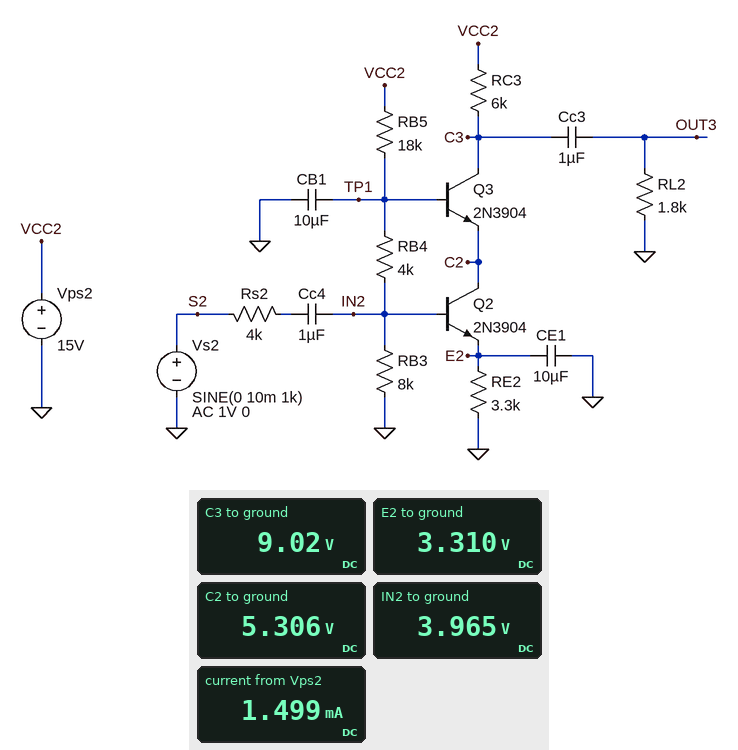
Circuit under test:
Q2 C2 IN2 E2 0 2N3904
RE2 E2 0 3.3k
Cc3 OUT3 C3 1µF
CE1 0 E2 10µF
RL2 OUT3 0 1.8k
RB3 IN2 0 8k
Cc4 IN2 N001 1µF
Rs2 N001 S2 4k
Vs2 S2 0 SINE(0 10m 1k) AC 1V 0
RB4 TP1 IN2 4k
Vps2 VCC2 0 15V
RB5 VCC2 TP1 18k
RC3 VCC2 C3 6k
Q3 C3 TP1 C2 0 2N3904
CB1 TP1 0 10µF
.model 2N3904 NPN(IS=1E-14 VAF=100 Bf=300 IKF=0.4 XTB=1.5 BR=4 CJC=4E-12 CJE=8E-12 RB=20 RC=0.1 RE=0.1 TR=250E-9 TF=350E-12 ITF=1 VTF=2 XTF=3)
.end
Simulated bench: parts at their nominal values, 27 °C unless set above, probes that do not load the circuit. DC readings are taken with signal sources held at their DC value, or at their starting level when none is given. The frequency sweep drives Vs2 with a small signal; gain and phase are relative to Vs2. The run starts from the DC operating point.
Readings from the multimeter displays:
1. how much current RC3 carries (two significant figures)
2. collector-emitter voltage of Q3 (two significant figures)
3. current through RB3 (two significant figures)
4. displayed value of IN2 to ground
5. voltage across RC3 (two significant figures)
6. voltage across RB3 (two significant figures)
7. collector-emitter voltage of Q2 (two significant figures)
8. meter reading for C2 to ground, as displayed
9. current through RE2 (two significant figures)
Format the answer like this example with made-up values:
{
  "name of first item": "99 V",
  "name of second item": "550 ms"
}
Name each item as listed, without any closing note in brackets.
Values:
{
  "how much current RC3 carries": "1.0 mA",
  "collector-emitter voltage of Q3": "3.7 V",
  "current through RB3": "500 µA",
  "displayed value of IN2 to ground": "3.965 V",
  "voltage across RC3": "6.0 V",
  "voltage across RB3": "4.0 V",
  "collector-emitter voltage of Q2": "2.0 V",
  "meter reading for C2 to ground, as displayed": "5.306 V",
  "current through RE2": "1.0 mA"
}
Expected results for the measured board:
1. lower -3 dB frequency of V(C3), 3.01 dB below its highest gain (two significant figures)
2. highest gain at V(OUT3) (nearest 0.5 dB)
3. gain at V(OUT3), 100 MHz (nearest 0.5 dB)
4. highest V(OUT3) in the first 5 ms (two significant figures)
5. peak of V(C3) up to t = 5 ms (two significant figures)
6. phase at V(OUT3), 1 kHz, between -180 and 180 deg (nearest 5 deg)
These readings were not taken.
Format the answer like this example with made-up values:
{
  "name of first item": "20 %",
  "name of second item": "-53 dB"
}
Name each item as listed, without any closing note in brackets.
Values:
{
  "lower -3 dB frequency of V(C3), 3.01 dB below its highest gain": "500 Hz",
  "highest gain at V(OUT3)": "25.0 dB",
  "gain at V(OUT3), 100 MHz": "-12.0 dB",
  "highest V(OUT3) in the first 5 ms": "160 mV",
  "peak of V(C3) up to t = 5 ms": "9.2 V",
  "phase at V(OUT3), 1 kHz, between -180 and 180 deg": "-150 deg"
}
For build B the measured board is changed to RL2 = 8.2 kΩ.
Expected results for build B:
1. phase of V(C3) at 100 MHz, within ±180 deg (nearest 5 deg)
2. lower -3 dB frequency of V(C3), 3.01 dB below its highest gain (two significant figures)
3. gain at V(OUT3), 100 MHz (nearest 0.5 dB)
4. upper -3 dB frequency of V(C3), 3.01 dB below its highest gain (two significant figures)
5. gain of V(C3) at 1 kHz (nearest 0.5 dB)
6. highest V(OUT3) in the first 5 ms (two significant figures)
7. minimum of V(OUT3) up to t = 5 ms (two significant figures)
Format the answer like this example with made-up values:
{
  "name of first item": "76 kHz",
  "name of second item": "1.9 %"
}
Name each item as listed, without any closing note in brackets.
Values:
{
  "phase of V(C3) at 100 MHz, within ±180 deg": "-15 deg",
  "lower -3 dB frequency of V(C3), 3.01 dB below its highest gain": "520 Hz",
  "gain at V(OUT3), 100 MHz": "-11.5 dB",
  "upper -3 dB frequency of V(C3), 3.01 dB below its highest gain": "3.6 MHz",
  "gain of V(C3) at 1 kHz": "32.0 dB",
  "highest V(OUT3) in the first 5 ms": "400 mV",
  "minimum of V(OUT3) up to t = 5 ms": "-400 mV"
}
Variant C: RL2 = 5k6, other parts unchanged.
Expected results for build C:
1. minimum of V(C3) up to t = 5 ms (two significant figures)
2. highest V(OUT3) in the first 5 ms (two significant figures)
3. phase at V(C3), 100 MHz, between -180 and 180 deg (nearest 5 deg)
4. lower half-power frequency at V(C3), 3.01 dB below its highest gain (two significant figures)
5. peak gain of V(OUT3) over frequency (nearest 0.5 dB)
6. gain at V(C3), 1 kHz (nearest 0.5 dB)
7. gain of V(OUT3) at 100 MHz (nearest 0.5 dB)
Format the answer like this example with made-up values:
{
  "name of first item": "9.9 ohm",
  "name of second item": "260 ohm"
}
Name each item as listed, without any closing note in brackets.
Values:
{
  "minimum of V(C3) up to t = 5 ms": "8.7 V",
  "highest V(OUT3) in the first 5 ms": "330 mV",
  "phase at V(C3), 100 MHz, between -180 and 180 deg": "-10 deg",
  "lower half-power frequency at V(C3), 3.01 dB below its highest gain": "520 Hz",
  "peak gain of V(OUT3) over frequency": "31.5 dB",
  "gain at V(C3), 1 kHz": "30.5 dB",
  "gain of V(OUT3) at 100 MHz": "-11.5 dB"
}
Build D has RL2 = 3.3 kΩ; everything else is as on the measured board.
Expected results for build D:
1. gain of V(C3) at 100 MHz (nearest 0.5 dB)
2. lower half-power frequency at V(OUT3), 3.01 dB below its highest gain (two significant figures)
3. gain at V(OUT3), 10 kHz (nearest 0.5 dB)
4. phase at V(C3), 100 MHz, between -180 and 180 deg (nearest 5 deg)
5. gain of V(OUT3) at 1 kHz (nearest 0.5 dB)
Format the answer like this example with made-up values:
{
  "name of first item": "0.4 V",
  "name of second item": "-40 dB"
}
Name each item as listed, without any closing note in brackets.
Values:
{
  "gain of V(C3) at 100 MHz": "-11.5 dB",
  "lower half-power frequency at V(OUT3), 3.01 dB below its highest gain": "520 Hz",
  "gain at V(OUT3), 10 kHz": "28.5 dB",
  "phase at V(C3), 100 MHz, between -180 and 180 deg": "-5 deg",
  "gain of V(OUT3) at 1 kHz": "27.5 dB"
}
